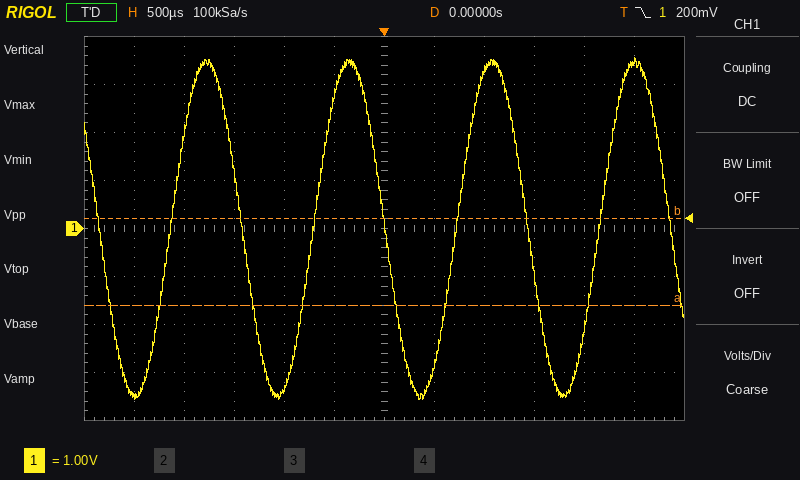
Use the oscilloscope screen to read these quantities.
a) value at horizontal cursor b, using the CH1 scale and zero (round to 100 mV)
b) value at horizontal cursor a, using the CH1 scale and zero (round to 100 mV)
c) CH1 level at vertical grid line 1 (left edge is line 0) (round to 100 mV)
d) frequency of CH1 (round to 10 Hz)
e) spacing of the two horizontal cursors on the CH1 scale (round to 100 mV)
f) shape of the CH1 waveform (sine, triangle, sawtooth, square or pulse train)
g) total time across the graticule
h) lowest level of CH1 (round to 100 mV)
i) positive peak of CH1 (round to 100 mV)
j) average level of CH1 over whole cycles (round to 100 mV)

200 mV
-1.6 V
-3.5 V
700 Hz
1.8 V
sine
6 ms
-3.6 V
3.6 V
0.0 V
